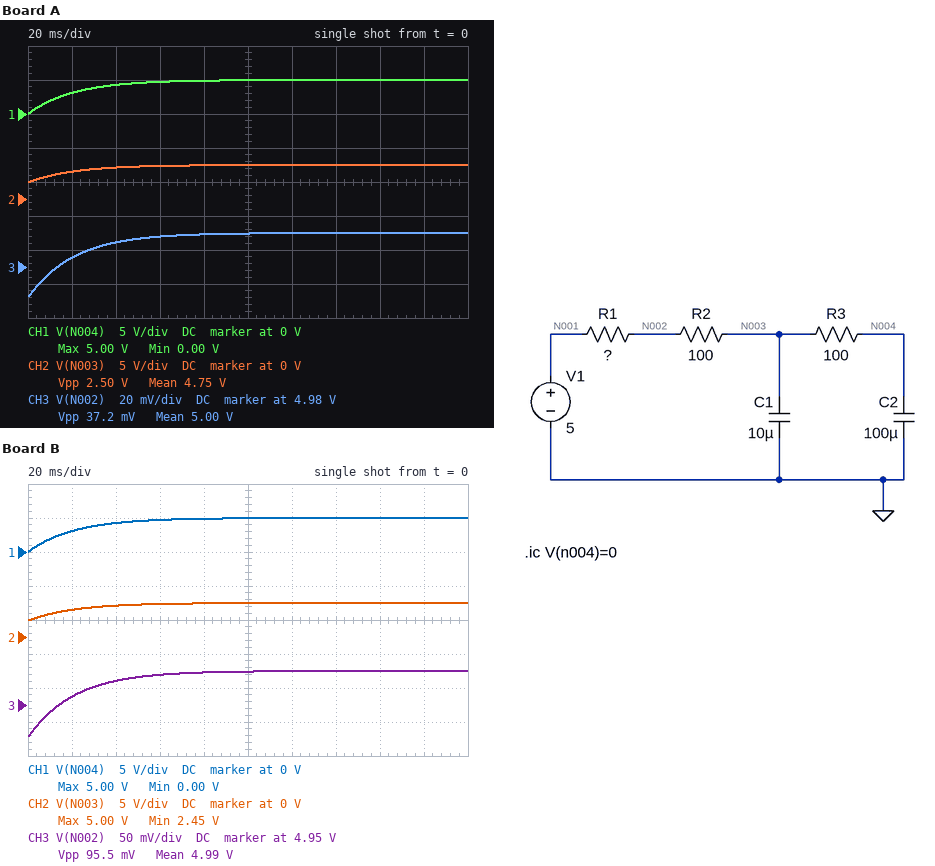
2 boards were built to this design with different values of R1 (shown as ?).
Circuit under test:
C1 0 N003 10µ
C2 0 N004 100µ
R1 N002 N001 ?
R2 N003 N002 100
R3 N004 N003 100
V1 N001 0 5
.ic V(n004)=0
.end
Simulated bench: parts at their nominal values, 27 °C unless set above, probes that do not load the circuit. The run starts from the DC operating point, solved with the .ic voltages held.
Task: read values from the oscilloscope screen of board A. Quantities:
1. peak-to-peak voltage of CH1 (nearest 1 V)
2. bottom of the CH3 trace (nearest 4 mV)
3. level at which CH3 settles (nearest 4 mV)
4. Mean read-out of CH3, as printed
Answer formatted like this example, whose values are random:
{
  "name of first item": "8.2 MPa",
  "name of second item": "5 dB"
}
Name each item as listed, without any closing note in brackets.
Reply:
{
  "peak-to-peak voltage of CH1": "5 V",
  "bottom of the CH3 trace": "4.964 V",
  "level at which CH3 settles": "5.000 V",
  "Mean read-out of CH3, as printed": "5.00 V"
}
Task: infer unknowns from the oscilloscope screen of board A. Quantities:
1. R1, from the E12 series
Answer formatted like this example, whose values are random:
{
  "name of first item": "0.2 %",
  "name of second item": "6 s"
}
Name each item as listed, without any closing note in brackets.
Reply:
{
  "R1, from the E12 series": "1.5 Ω"
}
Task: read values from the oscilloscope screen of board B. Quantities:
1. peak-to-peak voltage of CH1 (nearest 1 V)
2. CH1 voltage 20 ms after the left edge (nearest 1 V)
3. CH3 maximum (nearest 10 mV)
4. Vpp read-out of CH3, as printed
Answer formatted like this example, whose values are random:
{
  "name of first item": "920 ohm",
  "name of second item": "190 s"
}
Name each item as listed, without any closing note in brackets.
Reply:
{
  "peak-to-peak voltage of CH1": "5 V",
  "CH1 voltage 20 ms after the left edge": "3 V",
  "CH3 maximum": "5.00 V",
  "Vpp read-out of CH3, as printed": "95.5 mV"
}
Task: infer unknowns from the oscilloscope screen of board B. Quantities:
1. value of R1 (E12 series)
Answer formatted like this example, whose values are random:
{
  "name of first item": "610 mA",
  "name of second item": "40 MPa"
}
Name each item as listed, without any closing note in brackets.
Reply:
{
  "value of R1": "3.9 Ω"
}
